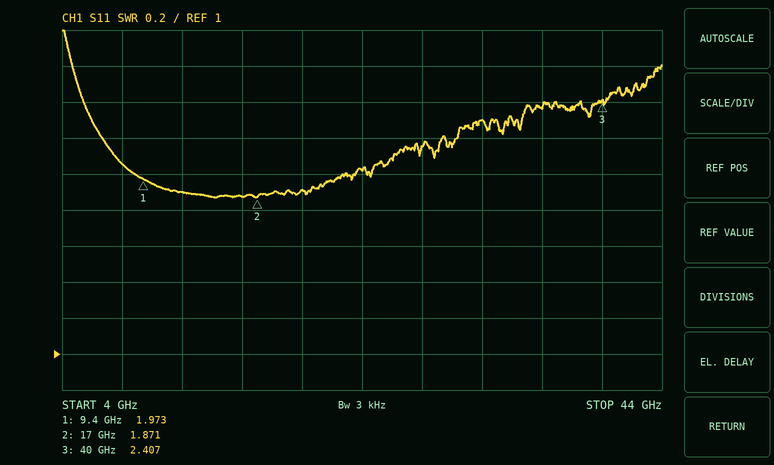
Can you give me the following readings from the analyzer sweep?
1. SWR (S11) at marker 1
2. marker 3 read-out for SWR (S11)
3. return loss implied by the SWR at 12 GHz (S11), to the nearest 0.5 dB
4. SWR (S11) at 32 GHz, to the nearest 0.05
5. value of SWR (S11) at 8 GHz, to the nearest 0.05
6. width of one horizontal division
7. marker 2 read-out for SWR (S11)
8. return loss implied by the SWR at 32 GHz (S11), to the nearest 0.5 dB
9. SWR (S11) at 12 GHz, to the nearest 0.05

1.973
2.407
10.0 dB
2.30
2.05
4 GHz
1.871
8.0 dB
1.90
